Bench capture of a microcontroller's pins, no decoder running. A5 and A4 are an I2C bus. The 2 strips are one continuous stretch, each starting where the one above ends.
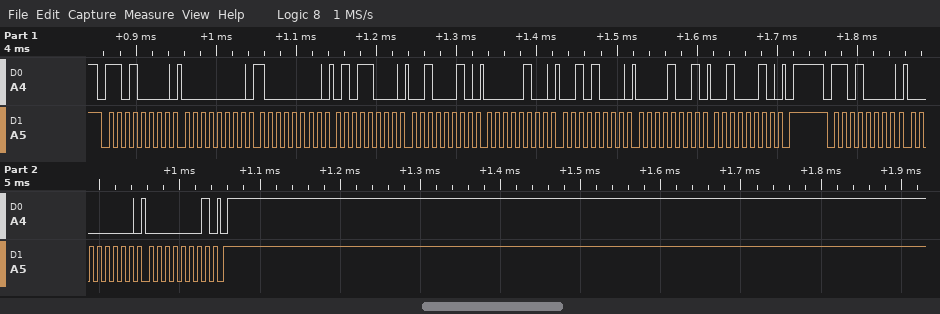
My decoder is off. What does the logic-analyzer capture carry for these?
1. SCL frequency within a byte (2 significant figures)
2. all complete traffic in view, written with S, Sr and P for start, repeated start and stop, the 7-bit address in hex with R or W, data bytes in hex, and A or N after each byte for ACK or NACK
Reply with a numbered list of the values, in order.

1. 100 kHz
2. S 68W A 00 A 80 A 58 A 22 A 04 A 28 A 09 A 22 A P S 68W A 00 A 01 A P
